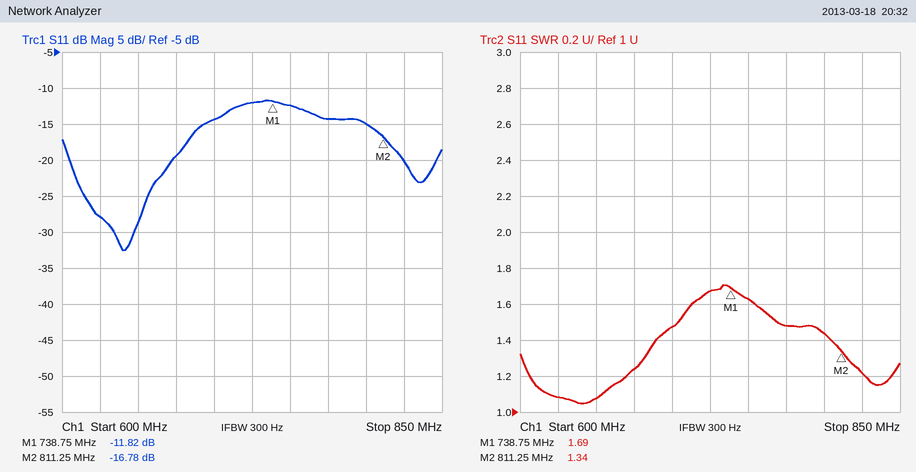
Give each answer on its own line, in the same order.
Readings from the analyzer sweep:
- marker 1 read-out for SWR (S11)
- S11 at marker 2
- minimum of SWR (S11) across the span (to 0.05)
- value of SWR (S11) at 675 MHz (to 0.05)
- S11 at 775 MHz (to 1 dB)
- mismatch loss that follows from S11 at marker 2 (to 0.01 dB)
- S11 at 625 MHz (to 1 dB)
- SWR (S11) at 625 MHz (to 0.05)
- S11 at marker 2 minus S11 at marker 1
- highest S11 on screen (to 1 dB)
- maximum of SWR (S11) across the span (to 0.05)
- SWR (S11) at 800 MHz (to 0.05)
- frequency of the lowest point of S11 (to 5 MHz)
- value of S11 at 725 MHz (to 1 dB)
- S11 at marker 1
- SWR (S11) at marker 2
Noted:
1.69
-16.78 dB
1.05
1.25
-14 dB
0.09 dB
-28 dB
1.10
-4.96 dB
-12 dB
1.70
1.45
640 MHz
-12 dB
-11.82 dB
1.34
